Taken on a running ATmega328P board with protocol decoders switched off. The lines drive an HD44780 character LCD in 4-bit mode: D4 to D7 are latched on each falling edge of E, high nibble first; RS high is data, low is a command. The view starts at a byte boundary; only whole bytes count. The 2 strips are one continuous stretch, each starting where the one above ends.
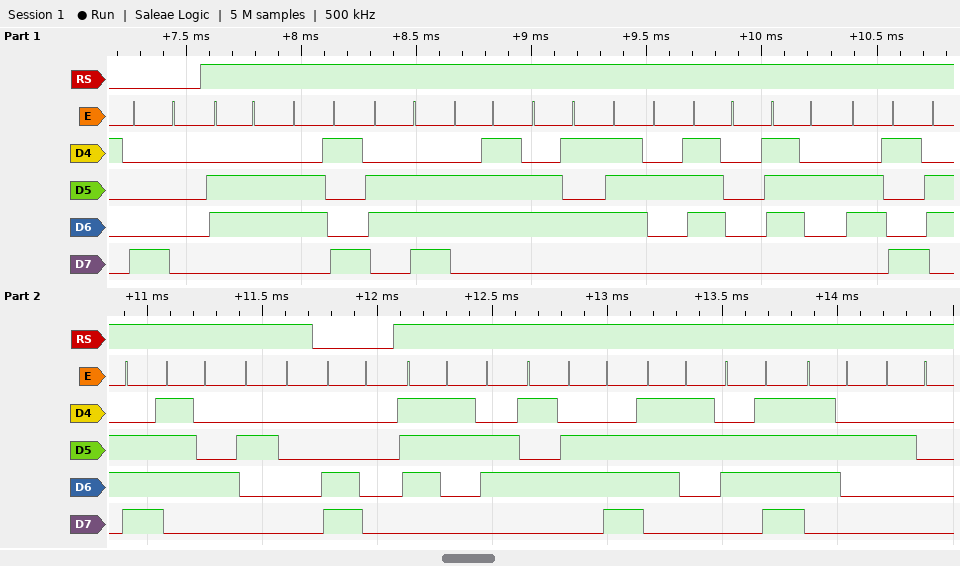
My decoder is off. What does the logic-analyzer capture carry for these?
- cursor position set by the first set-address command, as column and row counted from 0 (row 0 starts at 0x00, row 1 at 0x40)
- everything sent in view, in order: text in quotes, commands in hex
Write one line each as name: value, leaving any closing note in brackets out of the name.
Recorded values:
cursor position set by the first set-address command, as column and row counted from 0: column 0, row 0
everything sent in view, in order: text in quotes, commands in hex: 0x80 "fingerprint " 0xC0 "sensor "
